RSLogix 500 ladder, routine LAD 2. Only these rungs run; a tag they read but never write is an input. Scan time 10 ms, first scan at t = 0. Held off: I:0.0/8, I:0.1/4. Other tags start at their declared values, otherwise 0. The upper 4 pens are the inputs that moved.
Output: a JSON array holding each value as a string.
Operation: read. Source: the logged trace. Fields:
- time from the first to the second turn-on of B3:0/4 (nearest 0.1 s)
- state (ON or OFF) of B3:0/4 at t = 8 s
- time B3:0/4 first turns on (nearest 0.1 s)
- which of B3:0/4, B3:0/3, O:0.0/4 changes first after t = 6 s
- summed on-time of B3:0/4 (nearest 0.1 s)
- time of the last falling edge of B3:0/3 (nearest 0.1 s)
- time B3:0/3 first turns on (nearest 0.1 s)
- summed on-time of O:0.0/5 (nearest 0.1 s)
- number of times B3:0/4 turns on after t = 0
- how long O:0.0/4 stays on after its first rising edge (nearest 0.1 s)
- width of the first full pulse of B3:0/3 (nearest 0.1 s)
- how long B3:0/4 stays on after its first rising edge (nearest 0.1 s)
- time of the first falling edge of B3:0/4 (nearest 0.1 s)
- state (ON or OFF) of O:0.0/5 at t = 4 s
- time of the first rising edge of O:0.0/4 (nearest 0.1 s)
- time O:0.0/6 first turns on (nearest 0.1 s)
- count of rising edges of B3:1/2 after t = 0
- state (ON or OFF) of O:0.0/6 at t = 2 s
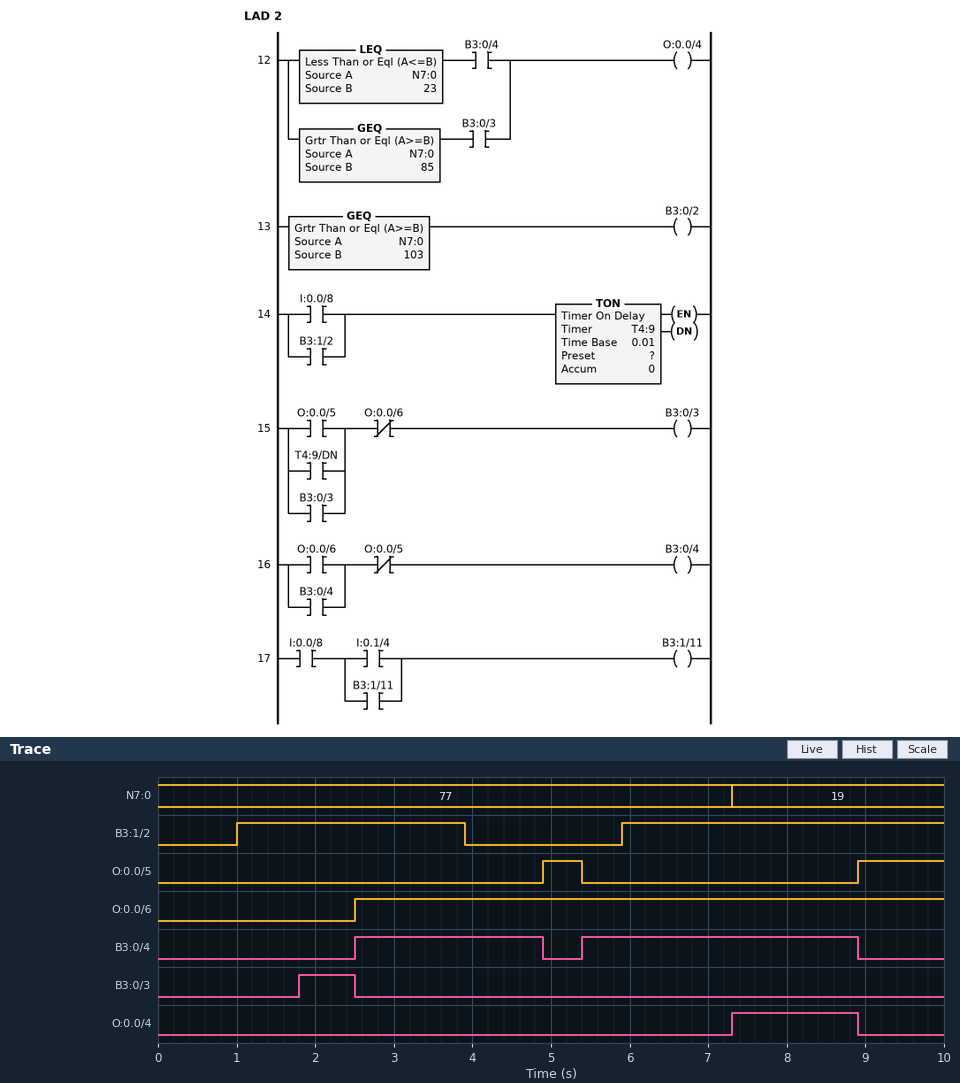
["2.9 s", "ON", "2.5 s", "O:0.0/4", "5.9 s", "2.5 s", "1.8 s", "1.6 s", "2", "1.6 s", "0.7 s", "2.4 s", "4.9 s", "OFF", "7.3 s", "2.5 s", "2", "OFF"]
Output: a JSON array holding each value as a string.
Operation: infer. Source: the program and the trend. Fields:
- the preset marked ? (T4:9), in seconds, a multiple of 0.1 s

["0.8 s"]
